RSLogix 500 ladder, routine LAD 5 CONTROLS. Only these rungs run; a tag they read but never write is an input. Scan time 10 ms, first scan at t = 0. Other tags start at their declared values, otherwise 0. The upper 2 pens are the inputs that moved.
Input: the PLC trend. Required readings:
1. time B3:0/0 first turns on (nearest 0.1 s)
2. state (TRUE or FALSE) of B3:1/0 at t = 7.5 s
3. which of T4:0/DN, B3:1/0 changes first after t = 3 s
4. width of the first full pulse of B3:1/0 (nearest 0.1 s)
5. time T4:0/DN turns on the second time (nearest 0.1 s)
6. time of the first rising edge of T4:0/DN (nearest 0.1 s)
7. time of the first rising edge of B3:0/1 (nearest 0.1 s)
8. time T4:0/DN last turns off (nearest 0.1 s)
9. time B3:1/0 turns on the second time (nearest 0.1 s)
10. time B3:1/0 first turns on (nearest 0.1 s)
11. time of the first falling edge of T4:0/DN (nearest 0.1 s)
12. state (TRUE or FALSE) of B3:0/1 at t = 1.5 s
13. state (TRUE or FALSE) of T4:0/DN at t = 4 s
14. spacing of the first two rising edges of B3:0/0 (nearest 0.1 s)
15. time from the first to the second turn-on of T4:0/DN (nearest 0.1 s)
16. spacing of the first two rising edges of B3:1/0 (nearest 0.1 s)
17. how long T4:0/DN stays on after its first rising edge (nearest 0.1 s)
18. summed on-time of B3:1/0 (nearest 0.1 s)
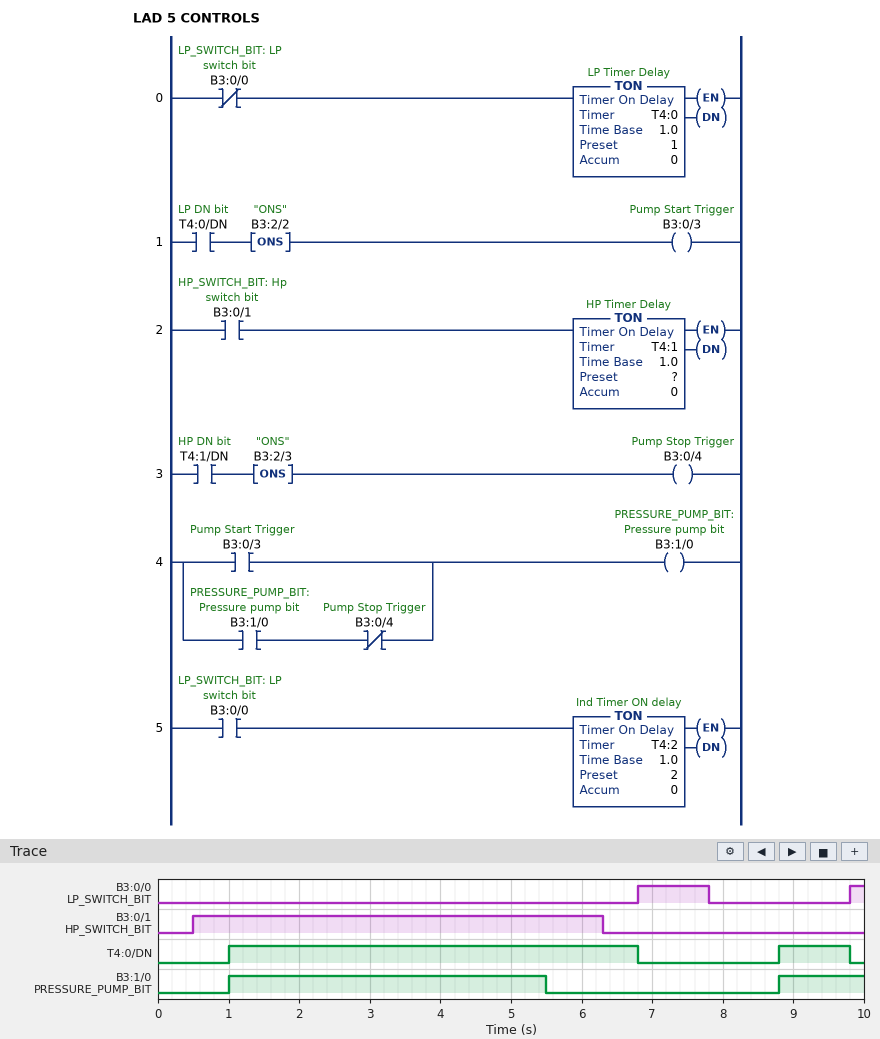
6.8 s
FALSE
B3:1/0
4.5 s
8.8 s
1.0 s
0.5 s
9.8 s
8.8 s
1.0 s
6.8 s
TRUE
TRUE
3.0 s
7.8 s
7.8 s
5.8 s
5.7 s
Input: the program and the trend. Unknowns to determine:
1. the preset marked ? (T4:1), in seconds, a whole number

5 s
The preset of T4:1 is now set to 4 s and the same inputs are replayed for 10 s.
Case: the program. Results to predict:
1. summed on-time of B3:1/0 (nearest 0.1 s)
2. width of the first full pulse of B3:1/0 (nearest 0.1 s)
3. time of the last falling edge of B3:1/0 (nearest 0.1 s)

4.7 s
3.5 s
4.5 s
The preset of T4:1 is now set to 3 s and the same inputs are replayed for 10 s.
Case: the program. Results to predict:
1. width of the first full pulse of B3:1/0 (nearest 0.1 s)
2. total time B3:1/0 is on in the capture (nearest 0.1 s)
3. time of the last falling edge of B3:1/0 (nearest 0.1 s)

2.5 s
3.7 s
3.5 s
